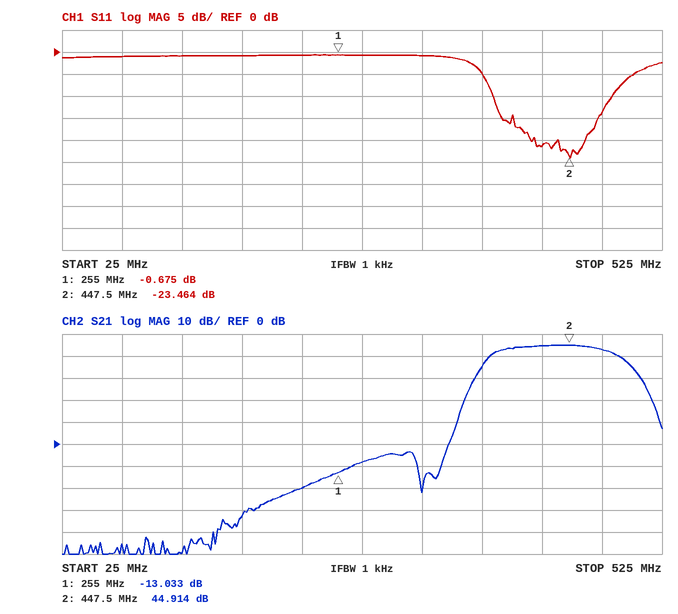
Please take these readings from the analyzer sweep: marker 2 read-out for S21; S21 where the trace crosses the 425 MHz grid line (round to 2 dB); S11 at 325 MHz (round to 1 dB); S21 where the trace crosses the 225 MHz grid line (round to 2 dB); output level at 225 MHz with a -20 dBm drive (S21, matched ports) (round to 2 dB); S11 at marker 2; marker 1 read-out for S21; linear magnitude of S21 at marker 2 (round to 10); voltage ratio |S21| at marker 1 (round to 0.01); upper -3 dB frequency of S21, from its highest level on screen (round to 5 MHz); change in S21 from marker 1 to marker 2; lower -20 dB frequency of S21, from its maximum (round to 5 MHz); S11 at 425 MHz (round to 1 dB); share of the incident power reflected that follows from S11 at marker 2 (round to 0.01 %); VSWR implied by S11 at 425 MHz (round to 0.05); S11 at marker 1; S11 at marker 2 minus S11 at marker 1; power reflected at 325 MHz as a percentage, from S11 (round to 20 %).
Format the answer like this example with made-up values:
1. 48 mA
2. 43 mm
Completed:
1. 44.914 dB
2. 44 dB
3. -1 dB
4. -20 dB
5. -40 dBm
6. -23.464 dB
7. -13.033 dB
8. 180
9. 0.22
10. 480 MHz
11. 57.947 dB
12. 365 MHz
13. -21 dB
14. 0.45 %
15. 1.20
16. -0.675 dB
17. -22.789 dB
18. 80 %
